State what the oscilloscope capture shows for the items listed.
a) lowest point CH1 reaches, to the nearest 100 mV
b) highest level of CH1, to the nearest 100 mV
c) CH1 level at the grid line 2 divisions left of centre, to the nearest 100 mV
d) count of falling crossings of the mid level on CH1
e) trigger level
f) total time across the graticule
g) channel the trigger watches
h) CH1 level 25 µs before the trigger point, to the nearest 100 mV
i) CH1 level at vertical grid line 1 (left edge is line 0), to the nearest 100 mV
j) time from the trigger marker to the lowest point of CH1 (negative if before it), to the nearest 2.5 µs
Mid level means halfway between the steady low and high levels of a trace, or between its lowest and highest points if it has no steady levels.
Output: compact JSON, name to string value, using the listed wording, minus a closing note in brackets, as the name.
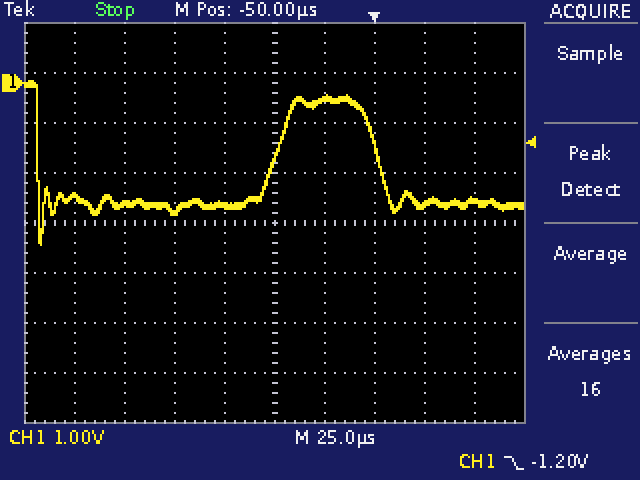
{"lowest point CH1 reaches, to the nearest 100 mV": "-3.2 V", "highest level of CH1, to the nearest 100 mV": "0.0 V", "CH1 level at the grid line 2 divisions left of centre, to the nearest 100 mV": "-2.6 V", "count of falling crossings of the mid level on CH1": "2", "trigger level": "-1.20 V", "total time across the graticule": "250 µs", "channel the trigger watches": "CH1", "CH1 level 25 µs before the trigger point, to the nearest 100 mV": "-300 mV", "CH1 level at vertical grid line 1 (left edge is line 0), to the nearest 100 mV": "-2.3 V", "time from the trigger marker to the lowest point of CH1 (negative if before it), to the nearest 2.5 µs": "-167.5 µs"}
